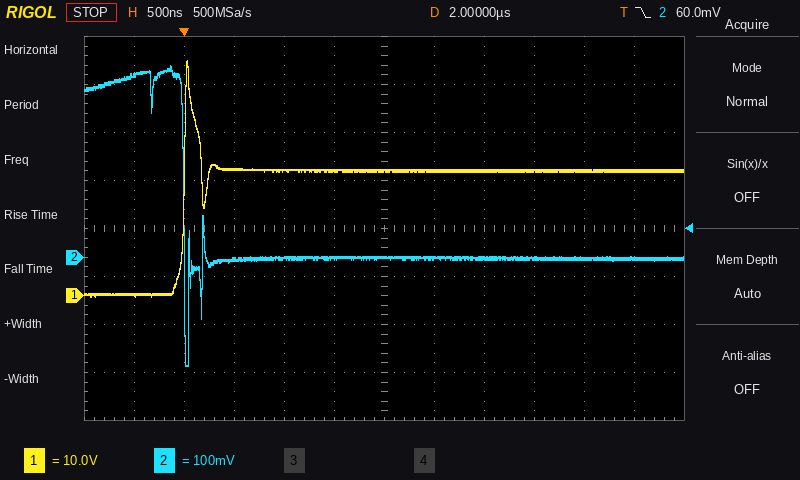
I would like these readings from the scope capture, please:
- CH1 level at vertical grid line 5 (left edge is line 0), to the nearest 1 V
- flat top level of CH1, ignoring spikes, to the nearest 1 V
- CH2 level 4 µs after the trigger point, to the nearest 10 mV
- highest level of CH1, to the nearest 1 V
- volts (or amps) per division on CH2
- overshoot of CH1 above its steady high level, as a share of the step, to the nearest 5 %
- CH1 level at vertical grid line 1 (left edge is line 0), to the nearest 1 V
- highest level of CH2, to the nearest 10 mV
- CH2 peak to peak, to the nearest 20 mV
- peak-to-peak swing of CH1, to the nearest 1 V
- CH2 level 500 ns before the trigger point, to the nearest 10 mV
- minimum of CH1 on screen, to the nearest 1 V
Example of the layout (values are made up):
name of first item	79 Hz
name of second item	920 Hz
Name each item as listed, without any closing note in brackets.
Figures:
CH1 level at vertical grid line 5 (left edge is line 0), to the nearest 1 V	26 V
flat top level of CH1, ignoring spikes, to the nearest 1 V	26 V
CH2 level 4 µs after the trigger point, to the nearest 10 mV	0 mV
highest level of CH1, to the nearest 1 V	49 V
volts (or amps) per division on CH2	100 mV
overshoot of CH1 above its steady high level, as a share of the step, to the nearest 5 %	90 %
CH1 level at vertical grid line 1 (left edge is line 0), to the nearest 1 V	0 V
highest level of CH2, to the nearest 10 mV	400 mV
CH2 peak to peak, to the nearest 20 mV	620 mV
peak-to-peak swing of CH1, to the nearest 1 V	49 V
CH2 level 500 ns before the trigger point, to the nearest 10 mV	380 mV
minimum of CH1 on screen, to the nearest 1 V	0 V
